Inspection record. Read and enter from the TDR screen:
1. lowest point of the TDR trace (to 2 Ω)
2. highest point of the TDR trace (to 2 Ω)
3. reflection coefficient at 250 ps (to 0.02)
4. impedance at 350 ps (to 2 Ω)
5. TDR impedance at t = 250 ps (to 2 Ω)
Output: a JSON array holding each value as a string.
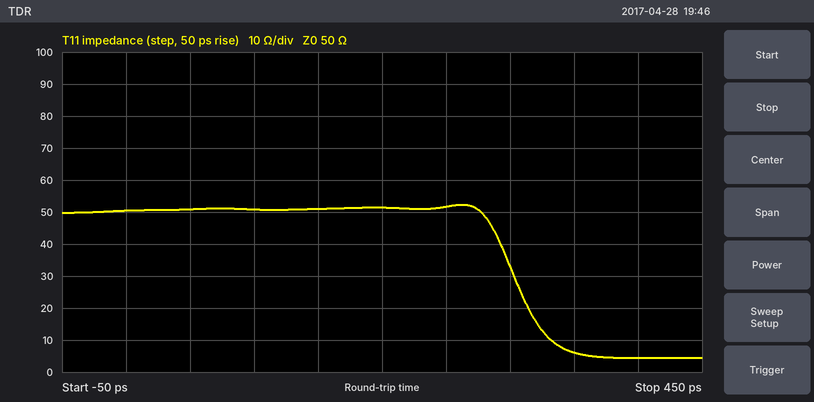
["4 Ω", "52 Ω", "+0.02", "6 Ω", "52 Ω"]
